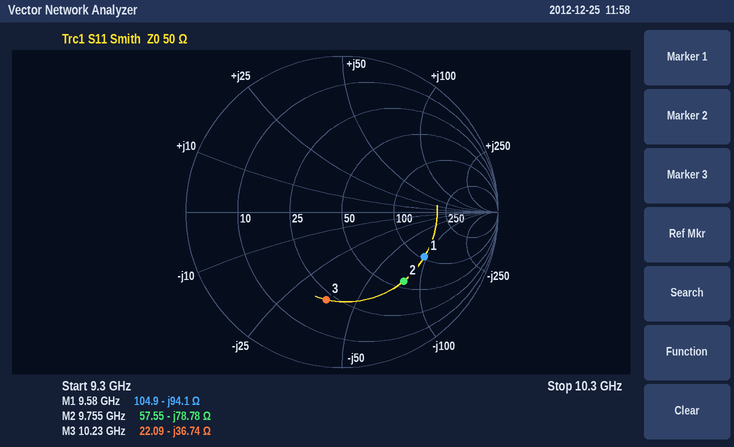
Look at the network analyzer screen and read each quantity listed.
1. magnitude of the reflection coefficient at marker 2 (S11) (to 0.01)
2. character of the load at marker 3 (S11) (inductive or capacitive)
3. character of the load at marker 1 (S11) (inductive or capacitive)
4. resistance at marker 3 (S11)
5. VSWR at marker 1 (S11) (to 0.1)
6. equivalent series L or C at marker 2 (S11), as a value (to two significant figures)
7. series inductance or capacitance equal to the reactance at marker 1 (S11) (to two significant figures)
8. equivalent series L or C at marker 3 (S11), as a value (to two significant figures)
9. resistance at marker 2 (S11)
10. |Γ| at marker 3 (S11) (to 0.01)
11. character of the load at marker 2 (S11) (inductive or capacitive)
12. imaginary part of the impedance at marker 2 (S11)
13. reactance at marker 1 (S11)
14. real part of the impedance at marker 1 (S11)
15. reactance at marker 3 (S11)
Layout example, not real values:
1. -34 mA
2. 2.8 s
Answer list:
1. 0.59
2. capacitive
3. capacitive
4. 22.09 Ω
5. 4.0
6. 210 fF
7. 180 fF
8. 420 fF
9. 57.55 Ω
10. 0.57
11. capacitive
12. -78.78 Ω
13. -94.1 Ω
14. 104.9 Ω
15. -36.74 Ω
